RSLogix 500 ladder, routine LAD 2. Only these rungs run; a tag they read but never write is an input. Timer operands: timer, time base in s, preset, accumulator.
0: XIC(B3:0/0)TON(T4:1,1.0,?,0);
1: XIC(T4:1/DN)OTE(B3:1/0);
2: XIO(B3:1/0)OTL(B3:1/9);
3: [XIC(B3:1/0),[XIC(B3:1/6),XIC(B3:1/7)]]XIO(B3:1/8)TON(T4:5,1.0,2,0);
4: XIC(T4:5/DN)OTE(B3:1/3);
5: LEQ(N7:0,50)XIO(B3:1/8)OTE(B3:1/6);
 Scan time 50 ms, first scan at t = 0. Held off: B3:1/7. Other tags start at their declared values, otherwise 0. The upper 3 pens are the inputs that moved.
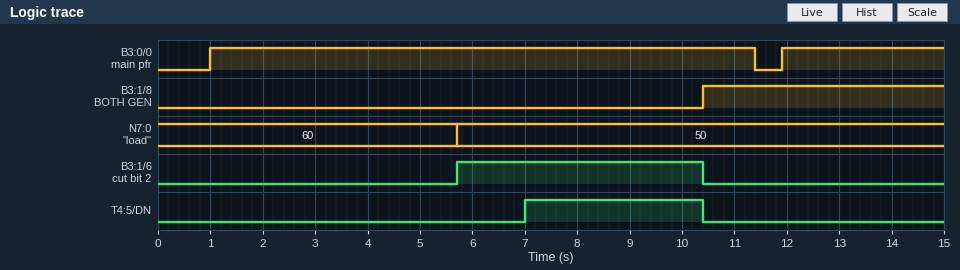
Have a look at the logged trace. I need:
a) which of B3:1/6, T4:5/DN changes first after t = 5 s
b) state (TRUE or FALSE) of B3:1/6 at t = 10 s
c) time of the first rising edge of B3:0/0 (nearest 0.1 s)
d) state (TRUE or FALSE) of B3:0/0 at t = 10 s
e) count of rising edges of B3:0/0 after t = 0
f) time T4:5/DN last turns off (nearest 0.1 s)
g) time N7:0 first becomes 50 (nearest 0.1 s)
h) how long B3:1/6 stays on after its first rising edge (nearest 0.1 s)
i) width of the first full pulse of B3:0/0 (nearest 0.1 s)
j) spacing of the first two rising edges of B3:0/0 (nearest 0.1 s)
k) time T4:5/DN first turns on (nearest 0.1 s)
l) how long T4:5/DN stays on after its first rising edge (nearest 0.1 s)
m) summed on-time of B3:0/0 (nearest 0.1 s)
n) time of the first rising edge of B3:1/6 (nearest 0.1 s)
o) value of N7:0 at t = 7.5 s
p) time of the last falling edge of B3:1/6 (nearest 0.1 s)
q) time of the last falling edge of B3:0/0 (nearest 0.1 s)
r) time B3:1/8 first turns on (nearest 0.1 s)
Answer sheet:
B3:1/6
TRUE
1.0 s
TRUE
2
10.4 s
5.7 s
4.7 s
10.4 s
10.9 s
7.0 s
3.4 s
13.5 s
5.7 s
50
10.4 s
11.4 s
10.4 s
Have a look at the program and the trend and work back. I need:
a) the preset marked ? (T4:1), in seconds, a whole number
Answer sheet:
4 s
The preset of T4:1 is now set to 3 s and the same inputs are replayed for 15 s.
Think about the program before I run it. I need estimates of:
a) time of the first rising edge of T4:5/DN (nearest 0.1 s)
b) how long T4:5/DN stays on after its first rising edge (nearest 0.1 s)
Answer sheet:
6.0 s
4.4 s
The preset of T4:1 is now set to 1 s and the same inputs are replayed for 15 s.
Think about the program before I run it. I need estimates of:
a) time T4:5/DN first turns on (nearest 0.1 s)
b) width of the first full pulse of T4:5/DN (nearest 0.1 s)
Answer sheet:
4.0 s
6.4 s
